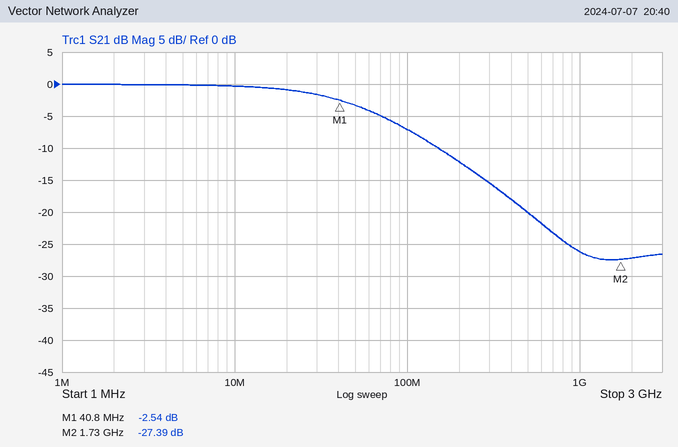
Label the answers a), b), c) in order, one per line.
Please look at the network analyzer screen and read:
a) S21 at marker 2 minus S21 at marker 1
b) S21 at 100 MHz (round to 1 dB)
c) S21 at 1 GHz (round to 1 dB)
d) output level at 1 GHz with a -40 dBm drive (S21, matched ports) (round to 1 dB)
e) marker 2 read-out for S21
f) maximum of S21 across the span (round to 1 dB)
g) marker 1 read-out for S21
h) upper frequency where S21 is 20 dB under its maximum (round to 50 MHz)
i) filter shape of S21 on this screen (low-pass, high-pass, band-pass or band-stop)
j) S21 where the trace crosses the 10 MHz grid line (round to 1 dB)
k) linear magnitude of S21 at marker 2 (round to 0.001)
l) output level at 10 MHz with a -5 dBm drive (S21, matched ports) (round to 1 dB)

a) -24.85 dB
b) -7 dB
c) -26 dB
d) -66 dBm
e) -27.39 dB
f) 0 dB
g) -2.54 dB
h) 500 MHz
i) low-pass
j) 0 dB
k) 0.043
l) -5 dBm
